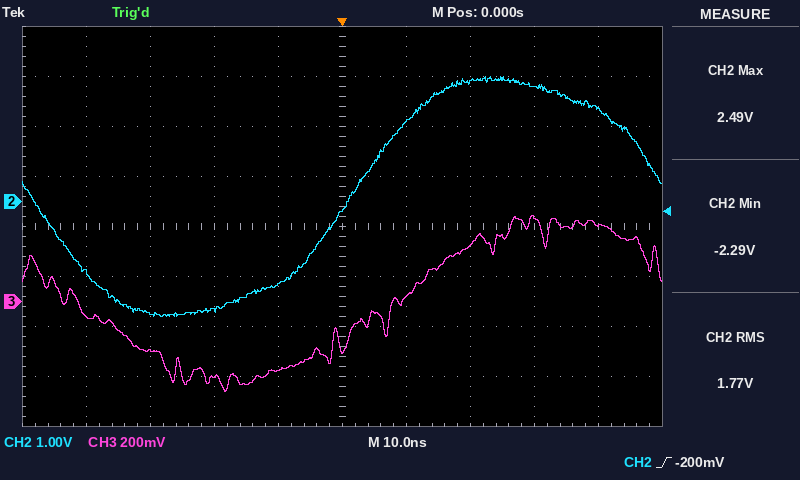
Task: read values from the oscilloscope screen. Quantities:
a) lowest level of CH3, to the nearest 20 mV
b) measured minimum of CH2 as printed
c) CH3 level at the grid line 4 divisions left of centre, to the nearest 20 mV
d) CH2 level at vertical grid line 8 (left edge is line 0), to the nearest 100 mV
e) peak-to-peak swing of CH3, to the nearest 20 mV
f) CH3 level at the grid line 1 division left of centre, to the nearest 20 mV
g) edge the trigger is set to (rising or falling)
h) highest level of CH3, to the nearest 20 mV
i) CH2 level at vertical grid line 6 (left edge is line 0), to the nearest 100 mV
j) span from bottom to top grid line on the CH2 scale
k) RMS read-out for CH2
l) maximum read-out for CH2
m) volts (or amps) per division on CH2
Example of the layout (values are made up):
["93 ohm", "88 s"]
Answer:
["-360 mV", "-2.29 V", "-60 mV", "2.3 V", "700 mV", "-280 mV", "rising", "340 mV", "1.6 V", "8 V", "1.77 V", "2.49 V", "1 V"]
